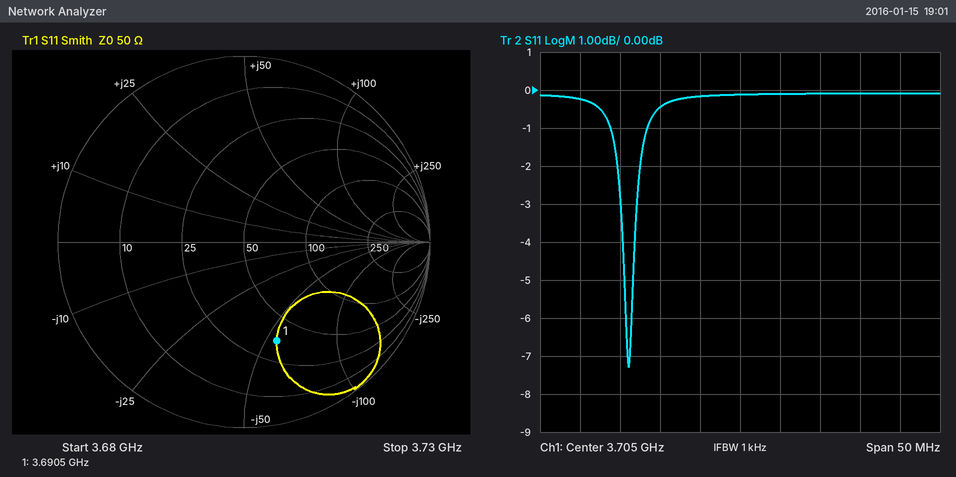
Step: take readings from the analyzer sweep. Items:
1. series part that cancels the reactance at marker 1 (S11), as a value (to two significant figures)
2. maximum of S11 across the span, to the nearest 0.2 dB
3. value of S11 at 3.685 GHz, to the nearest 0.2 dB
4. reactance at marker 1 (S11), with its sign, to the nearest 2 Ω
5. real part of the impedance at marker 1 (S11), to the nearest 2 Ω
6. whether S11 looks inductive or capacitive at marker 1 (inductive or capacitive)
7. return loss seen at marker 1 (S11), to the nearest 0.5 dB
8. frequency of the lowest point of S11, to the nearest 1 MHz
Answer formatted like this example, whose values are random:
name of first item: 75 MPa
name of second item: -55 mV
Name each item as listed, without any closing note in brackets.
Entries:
series part that cancels the reactance at marker 1 (S11), as a value: 2.4 nH
maximum of S11 across the span, to the nearest 0.2 dB: 0.0 dB
value of S11 at 3.685 GHz, to the nearest 0.2 dB: -0.2 dB
reactance at marker 1 (S11), with its sign, to the nearest 2 Ω: -56 Ω
real part of the impedance at marker 1 (S11), to the nearest 2 Ω: 36 Ω
whether S11 looks inductive or capacitive at marker 1: capacitive
return loss seen at marker 1 (S11), to the nearest 0.5 dB: 5.0 dB
frequency of the lowest point of S11, to the nearest 1 MHz: 3.691 GHz
